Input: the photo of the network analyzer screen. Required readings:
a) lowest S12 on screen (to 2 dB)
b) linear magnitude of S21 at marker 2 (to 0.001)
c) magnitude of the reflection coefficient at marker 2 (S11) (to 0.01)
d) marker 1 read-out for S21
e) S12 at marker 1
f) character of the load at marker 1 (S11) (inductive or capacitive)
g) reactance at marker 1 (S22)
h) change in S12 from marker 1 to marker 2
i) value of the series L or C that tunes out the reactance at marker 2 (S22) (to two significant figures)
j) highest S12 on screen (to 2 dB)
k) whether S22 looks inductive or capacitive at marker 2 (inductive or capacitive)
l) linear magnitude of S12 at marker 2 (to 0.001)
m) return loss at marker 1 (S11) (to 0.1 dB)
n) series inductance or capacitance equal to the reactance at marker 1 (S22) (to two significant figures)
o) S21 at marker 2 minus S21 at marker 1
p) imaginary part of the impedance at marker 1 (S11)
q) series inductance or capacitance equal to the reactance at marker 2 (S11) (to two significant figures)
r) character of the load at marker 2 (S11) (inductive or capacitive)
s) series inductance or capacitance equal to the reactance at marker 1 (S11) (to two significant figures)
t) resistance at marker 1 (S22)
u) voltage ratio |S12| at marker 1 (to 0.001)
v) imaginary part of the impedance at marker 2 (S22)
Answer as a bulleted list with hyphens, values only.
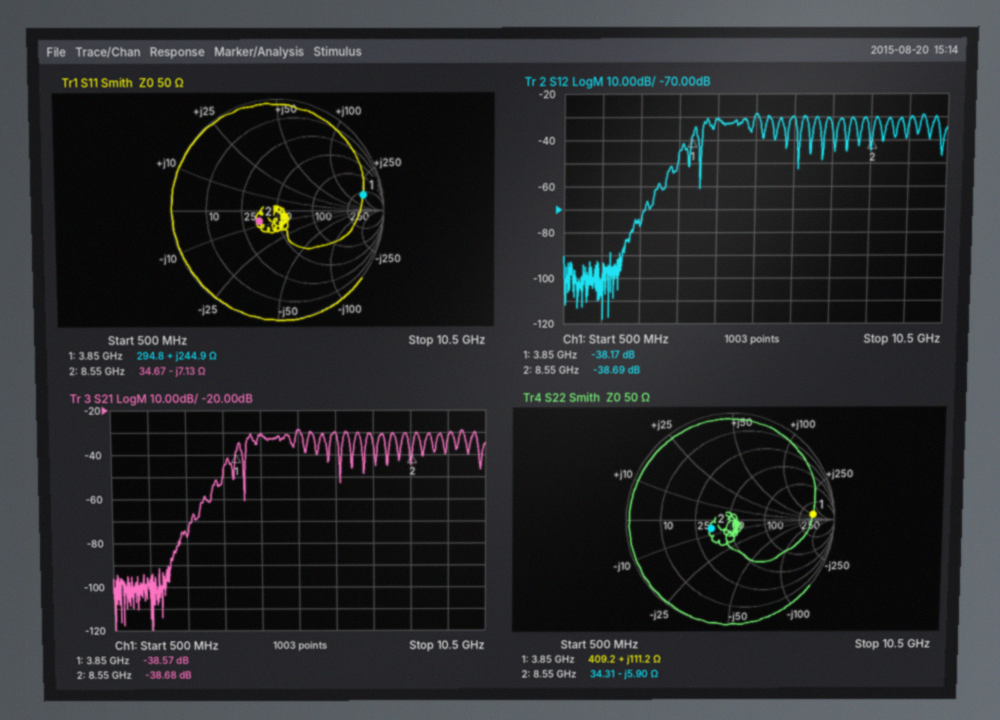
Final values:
- -118 dB
- 0.012
- 0.20
- -38.57 dB
- -38.17 dB
- inductive
- +111.2 Ω
- -0.52 dB
- 110 pH
- -28 dB
- capacitive
- 0.012
- 1.7 dB
- 4.6 nH
- -0.11 dB
- +244.9 Ω
- 2.6 pF
- capacitive
- 10 nH
- 409.2 Ω
- 0.012
- -5.90 Ω
